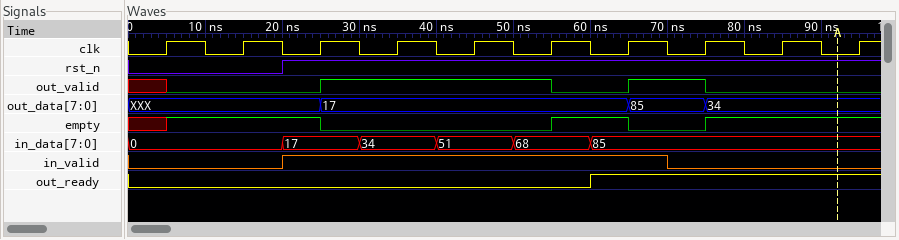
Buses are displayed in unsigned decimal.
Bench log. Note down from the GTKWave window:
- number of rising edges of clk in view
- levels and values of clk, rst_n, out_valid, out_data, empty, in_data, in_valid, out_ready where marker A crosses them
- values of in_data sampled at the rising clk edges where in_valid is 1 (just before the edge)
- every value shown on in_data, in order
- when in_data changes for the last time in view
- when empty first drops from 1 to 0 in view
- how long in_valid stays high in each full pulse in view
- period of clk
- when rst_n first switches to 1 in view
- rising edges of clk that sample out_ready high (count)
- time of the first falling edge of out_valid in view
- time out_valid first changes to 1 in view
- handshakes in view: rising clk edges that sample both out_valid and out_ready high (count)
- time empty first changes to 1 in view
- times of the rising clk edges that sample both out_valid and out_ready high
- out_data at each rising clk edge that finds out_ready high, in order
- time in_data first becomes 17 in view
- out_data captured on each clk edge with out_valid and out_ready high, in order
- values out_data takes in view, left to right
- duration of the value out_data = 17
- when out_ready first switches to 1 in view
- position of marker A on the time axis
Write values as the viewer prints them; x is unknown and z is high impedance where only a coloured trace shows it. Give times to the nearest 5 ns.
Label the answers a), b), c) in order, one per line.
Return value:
a) 10
b) clk=0, rst_n=1, out_valid=0, out_data=34, empty=1, in_data=85, in_valid=0, out_ready=1
c) 17, 34, 51, 68, 85
d) 0, 17, 34, 51, 68, 85
e) 60 ns
f) 25 ns
g) 50 ns
h) 10 ns
i) 20 ns
j) 4
k) 55 ns
l) 25 ns
m) 1
n) 5 ns
o) 75 ns
p) 17, 85, 34, 34
q) 20 ns
r) 85
s) XXX, 17, 85, 34
t) 40 ns
u) 60 ns
v) 90 ns
